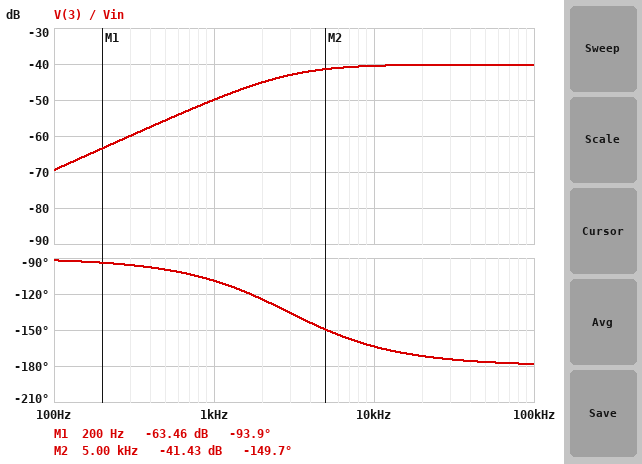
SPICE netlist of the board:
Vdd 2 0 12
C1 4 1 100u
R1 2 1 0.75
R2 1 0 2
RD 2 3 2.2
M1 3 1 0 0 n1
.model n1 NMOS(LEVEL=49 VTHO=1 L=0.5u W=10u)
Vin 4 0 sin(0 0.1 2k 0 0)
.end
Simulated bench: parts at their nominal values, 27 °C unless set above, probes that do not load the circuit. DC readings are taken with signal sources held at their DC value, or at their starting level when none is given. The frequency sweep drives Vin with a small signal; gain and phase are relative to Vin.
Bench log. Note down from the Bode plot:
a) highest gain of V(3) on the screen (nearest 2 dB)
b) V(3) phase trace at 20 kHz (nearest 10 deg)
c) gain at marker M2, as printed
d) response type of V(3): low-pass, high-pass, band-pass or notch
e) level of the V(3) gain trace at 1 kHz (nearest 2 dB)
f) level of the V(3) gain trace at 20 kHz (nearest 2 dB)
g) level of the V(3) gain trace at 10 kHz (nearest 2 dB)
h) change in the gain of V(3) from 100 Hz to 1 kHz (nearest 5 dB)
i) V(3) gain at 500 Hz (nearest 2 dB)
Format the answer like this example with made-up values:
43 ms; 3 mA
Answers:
-40 dB; -170 deg; -41.43 dB; high-pass; -50 dB; -40 dB; -40 dB; 20 dB; -56 dB
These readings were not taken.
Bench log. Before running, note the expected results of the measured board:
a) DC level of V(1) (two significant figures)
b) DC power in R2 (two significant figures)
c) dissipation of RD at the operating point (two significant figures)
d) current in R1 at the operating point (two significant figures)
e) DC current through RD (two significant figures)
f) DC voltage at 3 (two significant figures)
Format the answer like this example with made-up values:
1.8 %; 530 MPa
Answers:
8.7 V; 38 W; 9.6 mW; 4.4 A; 66 mA; 12 V
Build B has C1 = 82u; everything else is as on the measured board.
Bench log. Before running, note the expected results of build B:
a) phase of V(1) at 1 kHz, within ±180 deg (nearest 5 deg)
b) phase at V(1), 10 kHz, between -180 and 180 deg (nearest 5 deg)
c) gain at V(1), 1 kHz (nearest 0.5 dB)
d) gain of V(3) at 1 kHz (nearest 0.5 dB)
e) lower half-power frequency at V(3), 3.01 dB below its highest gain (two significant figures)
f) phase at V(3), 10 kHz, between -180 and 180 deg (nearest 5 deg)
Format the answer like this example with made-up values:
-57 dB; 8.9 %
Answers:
75 deg; 20 deg; -11.5 dB; -51.5 dB; 3.6 kHz; -160 deg
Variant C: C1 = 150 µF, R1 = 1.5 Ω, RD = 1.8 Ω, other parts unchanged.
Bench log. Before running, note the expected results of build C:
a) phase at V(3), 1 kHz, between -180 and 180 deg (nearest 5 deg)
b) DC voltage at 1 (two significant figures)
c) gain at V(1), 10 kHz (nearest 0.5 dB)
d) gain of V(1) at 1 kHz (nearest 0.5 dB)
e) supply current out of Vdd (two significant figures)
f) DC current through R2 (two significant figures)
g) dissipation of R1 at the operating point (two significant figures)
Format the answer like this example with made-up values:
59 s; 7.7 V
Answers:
-130 deg; 6.9 V; 0 dB; -4.0 dB; 3.5 A; 3.4 A; 18 W
